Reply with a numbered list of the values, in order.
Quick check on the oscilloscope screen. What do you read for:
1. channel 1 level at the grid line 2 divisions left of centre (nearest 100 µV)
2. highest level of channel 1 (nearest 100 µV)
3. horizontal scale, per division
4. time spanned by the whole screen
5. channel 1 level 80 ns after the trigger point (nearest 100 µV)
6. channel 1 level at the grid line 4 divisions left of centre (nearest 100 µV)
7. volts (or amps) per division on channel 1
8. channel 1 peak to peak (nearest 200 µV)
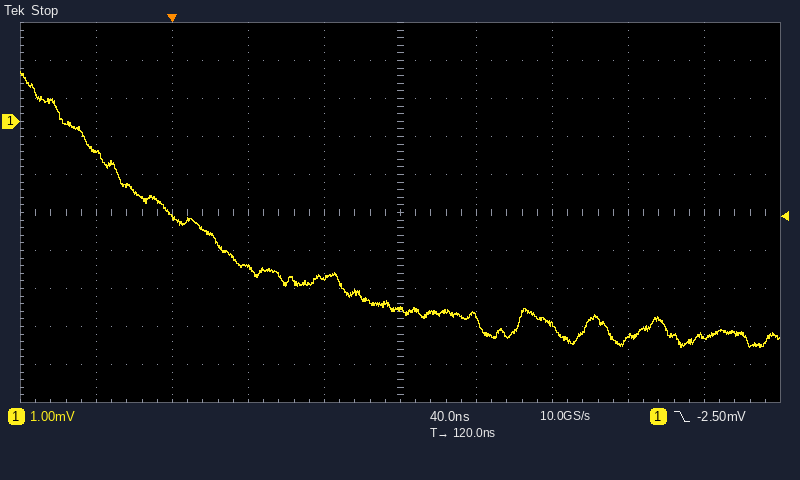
1. -3.9 mV
2. 1.3 mV
3. 40 ns
4. 400 ns
5. -4.1 mV
6. -800 µV
7. 1 mV
8. 7.2 mV
